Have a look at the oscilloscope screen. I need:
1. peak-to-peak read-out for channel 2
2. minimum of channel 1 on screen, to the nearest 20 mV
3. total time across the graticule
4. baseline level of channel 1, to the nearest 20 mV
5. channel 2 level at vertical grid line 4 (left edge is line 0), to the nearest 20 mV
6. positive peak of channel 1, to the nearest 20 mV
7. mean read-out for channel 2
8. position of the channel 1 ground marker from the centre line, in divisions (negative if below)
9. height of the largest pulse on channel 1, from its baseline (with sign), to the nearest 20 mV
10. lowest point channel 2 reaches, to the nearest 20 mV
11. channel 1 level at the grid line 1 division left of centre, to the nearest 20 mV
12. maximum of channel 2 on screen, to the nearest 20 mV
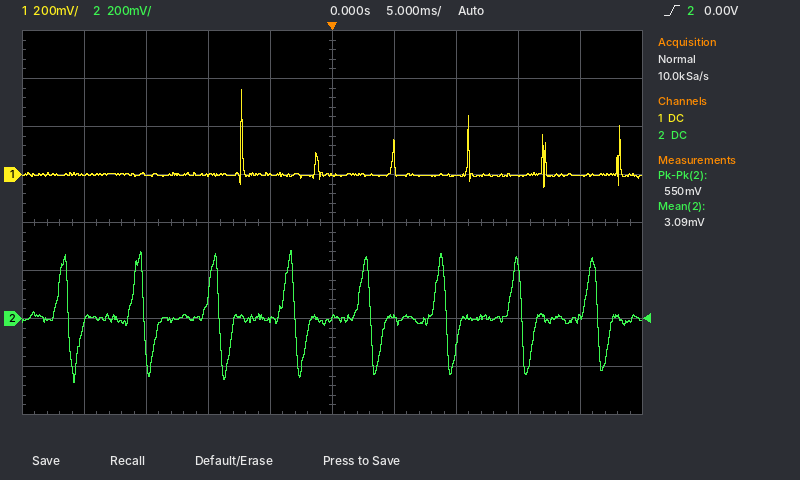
550 mV
-60 mV
50 ms
0 mV
0 mV
360 mV
3.09 mV
+1.0 div
+360 mV
-260 mV
0 mV
280 mV
